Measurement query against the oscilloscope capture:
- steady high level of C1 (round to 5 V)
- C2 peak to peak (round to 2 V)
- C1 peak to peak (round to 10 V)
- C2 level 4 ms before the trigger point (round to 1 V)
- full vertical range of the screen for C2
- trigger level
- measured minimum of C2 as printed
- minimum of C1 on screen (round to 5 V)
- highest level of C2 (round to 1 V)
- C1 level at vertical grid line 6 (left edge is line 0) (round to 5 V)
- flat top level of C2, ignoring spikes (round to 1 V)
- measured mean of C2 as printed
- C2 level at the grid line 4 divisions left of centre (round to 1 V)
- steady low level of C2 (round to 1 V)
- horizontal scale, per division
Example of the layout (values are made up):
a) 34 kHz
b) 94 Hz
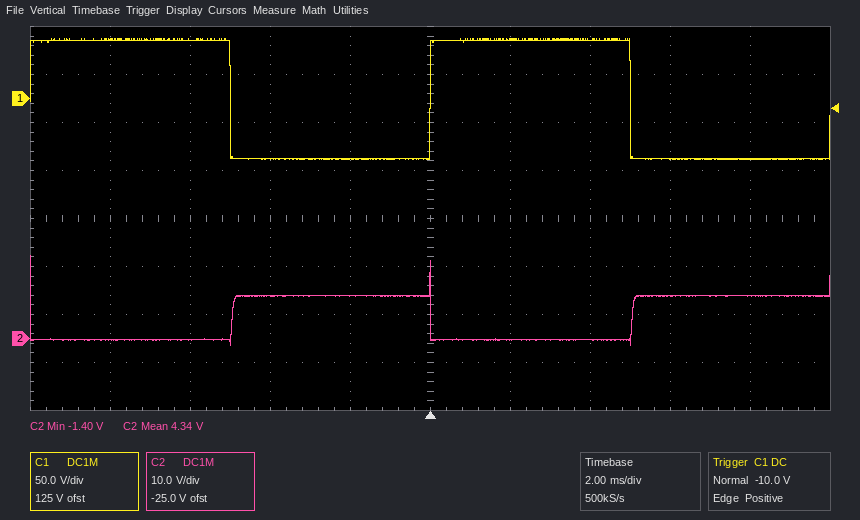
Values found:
a) 60 V
b) 18 V
c) 130 V
d) 9 V
e) 80 V
f) -10.0 V
g) -1.40 V
h) -65 V
i) 17 V
j) 60 V
k) 9 V
l) 4.34 V
m) 0 V
n) 0 V
o) 2 ms
